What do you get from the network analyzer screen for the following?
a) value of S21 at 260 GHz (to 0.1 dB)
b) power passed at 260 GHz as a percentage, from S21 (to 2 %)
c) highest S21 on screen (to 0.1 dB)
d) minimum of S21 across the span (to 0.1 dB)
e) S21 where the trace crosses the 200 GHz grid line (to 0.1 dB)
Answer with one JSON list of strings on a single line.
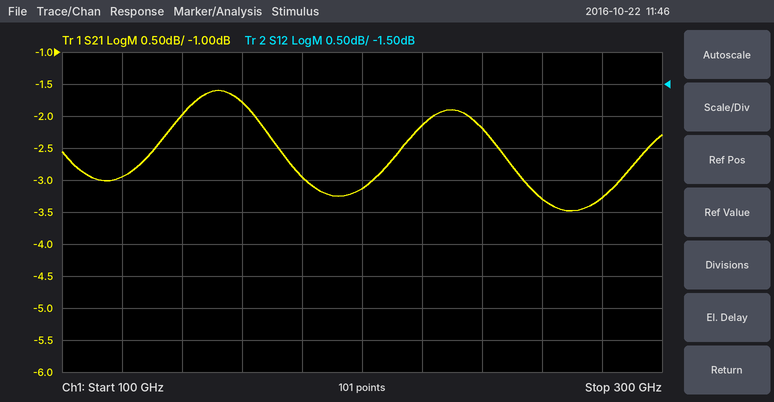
["-3.3 dB", "46 %", "-1.6 dB", "-3.5 dB", "-3.1 dB"]
